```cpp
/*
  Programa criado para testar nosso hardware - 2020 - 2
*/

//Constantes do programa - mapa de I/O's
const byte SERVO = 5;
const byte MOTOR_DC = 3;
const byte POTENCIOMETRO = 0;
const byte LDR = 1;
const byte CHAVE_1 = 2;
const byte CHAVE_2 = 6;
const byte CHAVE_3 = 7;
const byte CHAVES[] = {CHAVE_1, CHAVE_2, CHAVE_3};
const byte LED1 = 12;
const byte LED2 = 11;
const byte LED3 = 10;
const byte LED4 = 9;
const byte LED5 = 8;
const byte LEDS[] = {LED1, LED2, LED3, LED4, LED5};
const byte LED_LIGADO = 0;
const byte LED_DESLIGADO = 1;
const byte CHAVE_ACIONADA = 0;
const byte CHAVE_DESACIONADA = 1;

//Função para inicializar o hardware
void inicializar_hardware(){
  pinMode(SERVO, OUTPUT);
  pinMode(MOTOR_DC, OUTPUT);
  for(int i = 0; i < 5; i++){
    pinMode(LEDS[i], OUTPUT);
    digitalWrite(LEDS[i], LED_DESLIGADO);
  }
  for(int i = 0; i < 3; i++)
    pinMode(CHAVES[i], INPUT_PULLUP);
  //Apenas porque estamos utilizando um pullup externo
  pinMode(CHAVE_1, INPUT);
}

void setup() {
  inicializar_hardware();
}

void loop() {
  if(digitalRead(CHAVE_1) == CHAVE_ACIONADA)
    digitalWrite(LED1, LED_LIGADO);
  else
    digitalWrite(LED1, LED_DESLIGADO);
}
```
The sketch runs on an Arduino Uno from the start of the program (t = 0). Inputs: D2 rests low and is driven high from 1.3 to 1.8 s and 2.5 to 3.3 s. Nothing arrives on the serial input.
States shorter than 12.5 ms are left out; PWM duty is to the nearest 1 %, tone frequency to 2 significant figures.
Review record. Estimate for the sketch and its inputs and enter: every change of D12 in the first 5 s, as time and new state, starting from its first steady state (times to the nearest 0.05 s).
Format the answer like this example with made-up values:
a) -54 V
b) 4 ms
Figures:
a) 0 s low; 1.3 s high; 1.8 s low; 2.5 s high; 3.3 s low
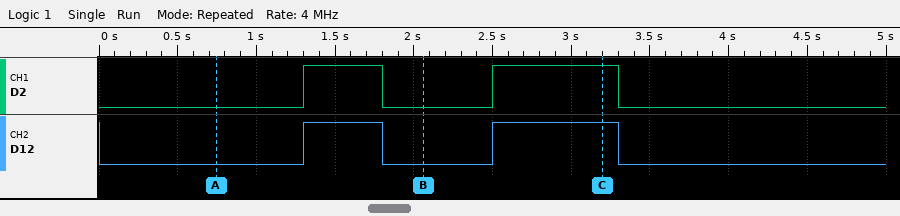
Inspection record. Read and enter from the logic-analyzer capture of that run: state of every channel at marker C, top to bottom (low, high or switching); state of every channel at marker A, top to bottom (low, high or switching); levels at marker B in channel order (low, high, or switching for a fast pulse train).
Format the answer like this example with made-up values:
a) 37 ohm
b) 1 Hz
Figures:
a) D2 high, D12 high
b) D2 low, D12 low
c) D2 low, D12 low
